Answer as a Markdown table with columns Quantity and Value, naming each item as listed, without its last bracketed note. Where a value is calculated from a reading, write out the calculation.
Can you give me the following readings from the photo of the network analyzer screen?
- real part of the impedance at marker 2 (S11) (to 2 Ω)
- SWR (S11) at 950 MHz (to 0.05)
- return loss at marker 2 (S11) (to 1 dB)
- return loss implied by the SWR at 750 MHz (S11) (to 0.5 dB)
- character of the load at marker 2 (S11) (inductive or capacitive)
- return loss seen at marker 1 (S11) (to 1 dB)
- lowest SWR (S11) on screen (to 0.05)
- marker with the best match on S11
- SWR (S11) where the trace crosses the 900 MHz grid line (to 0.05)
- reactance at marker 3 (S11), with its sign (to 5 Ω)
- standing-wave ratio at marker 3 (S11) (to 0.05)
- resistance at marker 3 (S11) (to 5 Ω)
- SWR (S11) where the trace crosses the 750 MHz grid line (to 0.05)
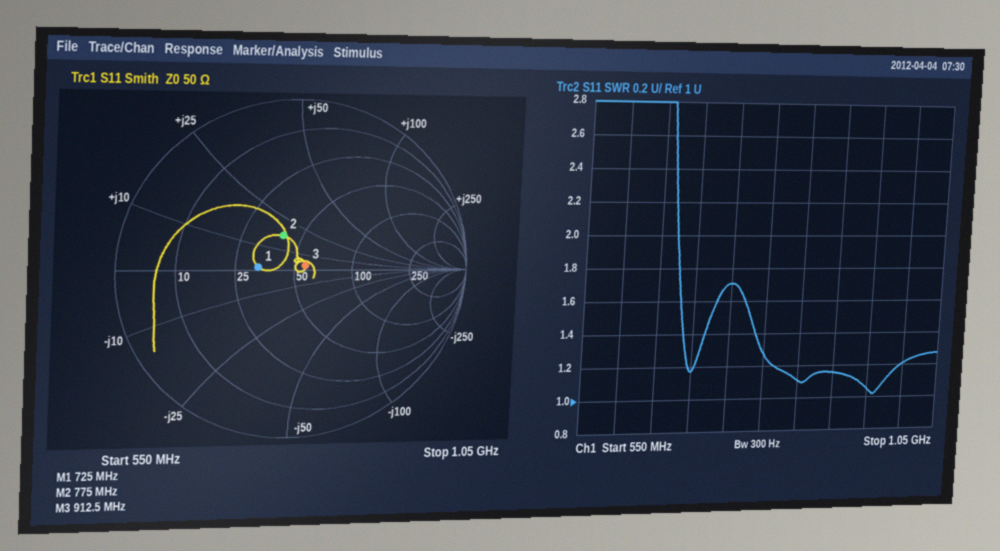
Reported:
| Quantity | Value |
|---|---|
| real part of the impedance at marker 2 (S11) | 40 Ω |
| SWR (S11) at 950 MHz | 1.05 |
| return loss at marker 2 (S11) | 13 dB |
| return loss implied by the SWR at 750 MHz (S11) | −20 log10((1.7 − 1)/(1.7 + 1)) ≈ 11.7 dB, so 11.5 dB to the nearest 0.5 dB |
| character of the load at marker 2 (S11) | inductive |
| return loss seen at marker 1 (S11) | 14 dB |
| lowest SWR (S11) on screen | 1.00 |
| marker with the best match on S11 | marker 3 |
| SWR (S11) where the trace crosses the 900 MHz grid line | 1.15 |
| reactance at marker 3 (S11), with its sign | +5 Ω |
| standing-wave ratio at marker 3 (S11) | 1.15 |
| resistance at marker 3 (S11) | 55 Ω |
| SWR (S11) where the trace crosses the 750 MHz grid line | 1.70 |
